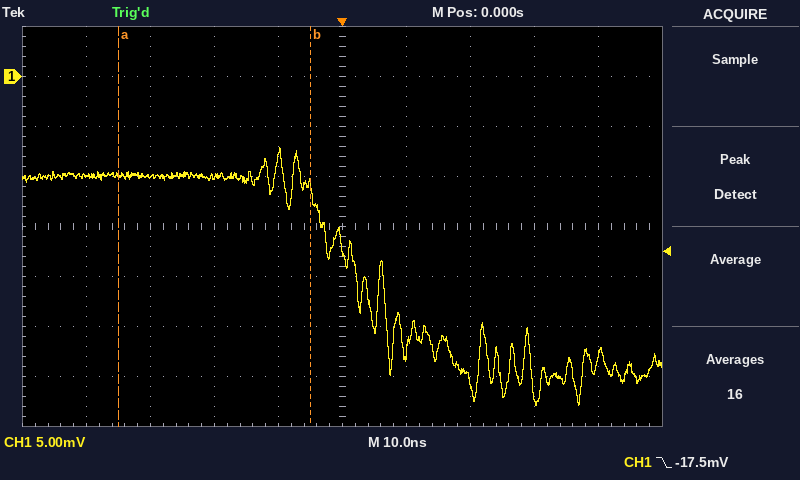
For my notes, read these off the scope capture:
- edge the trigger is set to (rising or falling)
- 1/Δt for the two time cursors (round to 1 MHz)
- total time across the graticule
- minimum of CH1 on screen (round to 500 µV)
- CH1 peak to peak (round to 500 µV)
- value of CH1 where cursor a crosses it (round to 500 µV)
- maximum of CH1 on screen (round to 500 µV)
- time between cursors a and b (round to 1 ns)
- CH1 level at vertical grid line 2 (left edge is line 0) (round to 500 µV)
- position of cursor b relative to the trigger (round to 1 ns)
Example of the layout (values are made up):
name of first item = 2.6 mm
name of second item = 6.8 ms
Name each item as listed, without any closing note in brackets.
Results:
edge the trigger is set to = falling
1/Δt for the two time cursors = 33 MHz
total time across the graticule = 100 ns
minimum of CH1 on screen = -33.0 mV
CH1 peak to peak = 26.0 mV
value of CH1 where cursor a crosses it = -10.0 mV
maximum of CH1 on screen = -7.0 mV
time between cursors a and b = 30 ns
CH1 level at vertical grid line 2 (left edge is line 0) = -10.0 mV
position of cursor b relative to the trigger = -5 ns
